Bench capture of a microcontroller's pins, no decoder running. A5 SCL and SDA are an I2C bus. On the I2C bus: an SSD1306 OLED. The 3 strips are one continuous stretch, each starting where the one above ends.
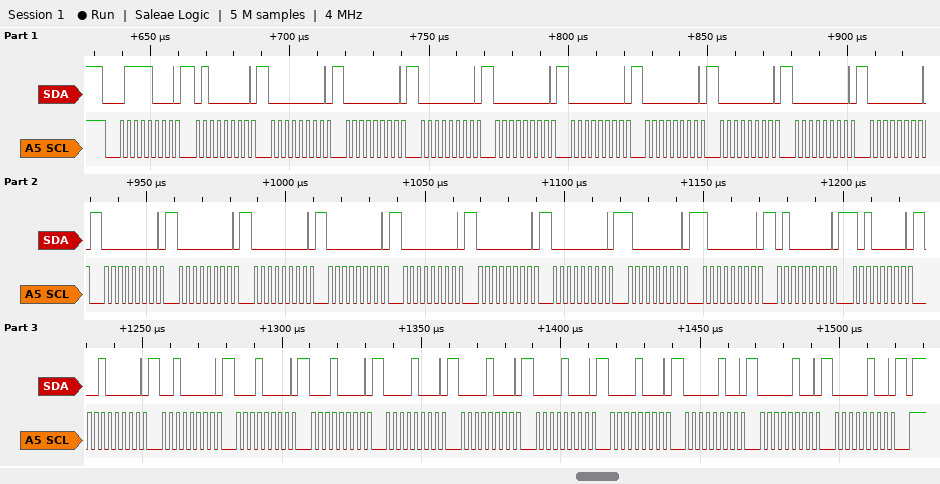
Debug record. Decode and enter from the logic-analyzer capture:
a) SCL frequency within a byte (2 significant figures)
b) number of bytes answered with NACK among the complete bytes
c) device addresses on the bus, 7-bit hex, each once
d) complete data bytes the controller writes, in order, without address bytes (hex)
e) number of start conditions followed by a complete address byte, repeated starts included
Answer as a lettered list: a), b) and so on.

a) 400 kHz
b) 0
c) 0x3C
d) 40 00 00 00 00 00 00 00 00 00 00 00 00 00 00 00 00 80 80 40 A0 20 20 10 10 08 08 08 08 04 04 04
e) 1
